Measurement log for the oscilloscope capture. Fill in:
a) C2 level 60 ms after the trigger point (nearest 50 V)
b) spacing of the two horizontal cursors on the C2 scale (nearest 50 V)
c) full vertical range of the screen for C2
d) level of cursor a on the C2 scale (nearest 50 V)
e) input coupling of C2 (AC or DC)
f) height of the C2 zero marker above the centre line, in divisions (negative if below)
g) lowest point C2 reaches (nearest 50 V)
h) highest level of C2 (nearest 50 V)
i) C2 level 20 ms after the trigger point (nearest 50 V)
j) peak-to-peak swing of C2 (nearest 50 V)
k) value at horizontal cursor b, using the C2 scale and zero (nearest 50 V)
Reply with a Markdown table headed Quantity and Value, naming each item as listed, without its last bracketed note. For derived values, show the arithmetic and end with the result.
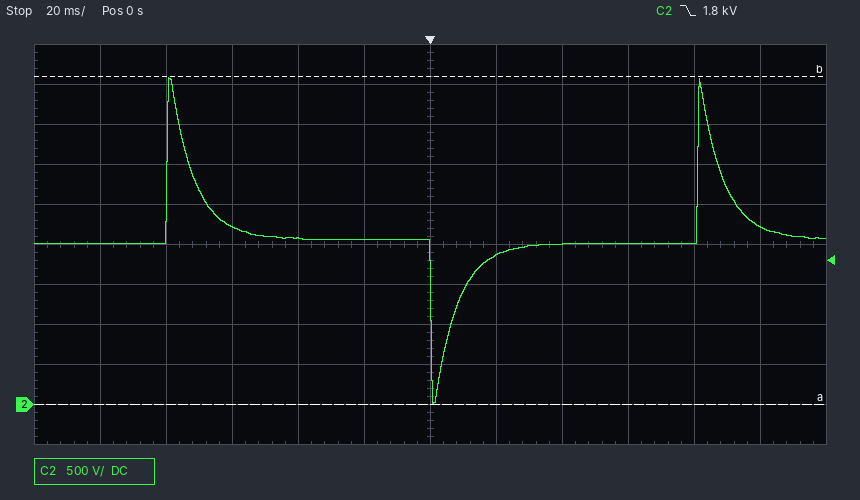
| Quantity | Value |
|---|---|
| C2 level 60 ms after the trigger point | 2.00 kV |
| spacing of the two horizontal cursors on the C2 scale | 4.10 kV |
| full vertical range of the screen for C2 | 5 kV |
| level of cursor a on the C2 scale | 0 V |
| input coupling of C2 | DC |
| height of the C2 zero marker above the centre line, in divisions | -4.0 div |
| lowest point C2 reaches | 0 V |
| highest level of C2 | 4.10 kV |
| C2 level 20 ms after the trigger point | 1.85 kV |
| peak-to-peak swing of C2 | 4.10 kV − (0 V) = 4.10 kV |
| value at horizontal cursor b, using the C2 scale and zero | 4.10 kV |
